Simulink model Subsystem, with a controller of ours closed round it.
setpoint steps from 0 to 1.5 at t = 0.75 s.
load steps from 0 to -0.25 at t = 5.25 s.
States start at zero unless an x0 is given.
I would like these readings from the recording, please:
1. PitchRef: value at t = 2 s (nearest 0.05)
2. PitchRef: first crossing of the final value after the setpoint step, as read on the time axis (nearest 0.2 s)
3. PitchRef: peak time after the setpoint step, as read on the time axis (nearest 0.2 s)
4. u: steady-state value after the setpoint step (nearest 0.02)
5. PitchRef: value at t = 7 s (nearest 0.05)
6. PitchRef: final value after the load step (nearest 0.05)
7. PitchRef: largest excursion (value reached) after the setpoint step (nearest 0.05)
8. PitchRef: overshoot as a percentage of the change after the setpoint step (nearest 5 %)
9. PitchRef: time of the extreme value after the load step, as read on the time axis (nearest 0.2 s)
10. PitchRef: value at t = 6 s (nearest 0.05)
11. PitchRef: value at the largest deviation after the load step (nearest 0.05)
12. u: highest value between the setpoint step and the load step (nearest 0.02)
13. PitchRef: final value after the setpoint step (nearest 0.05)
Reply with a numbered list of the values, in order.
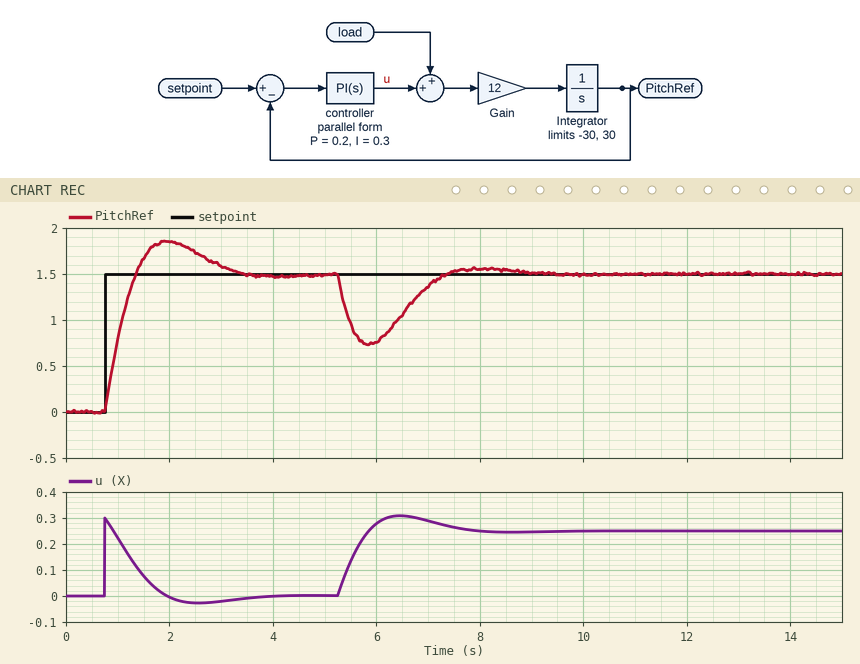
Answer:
1. 1.85
2. 1.4 s
3. 2.0 s
4. 0.00
5. 1.35
6. 1.50
7. 1.85
8. 25 %
9. 5.8 s
10. 0.75
11. 0.75
12. 0.30
13. 1.50
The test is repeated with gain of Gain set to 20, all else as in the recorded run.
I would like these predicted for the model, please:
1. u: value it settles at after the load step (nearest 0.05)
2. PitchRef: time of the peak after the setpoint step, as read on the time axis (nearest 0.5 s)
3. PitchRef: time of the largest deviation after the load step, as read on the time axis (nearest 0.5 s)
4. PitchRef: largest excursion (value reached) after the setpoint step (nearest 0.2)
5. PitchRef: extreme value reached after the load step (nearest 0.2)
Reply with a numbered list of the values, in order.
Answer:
1. 0.25
2. 1.5 s
3. 5.5 s
4. 1.8
5. 0.6
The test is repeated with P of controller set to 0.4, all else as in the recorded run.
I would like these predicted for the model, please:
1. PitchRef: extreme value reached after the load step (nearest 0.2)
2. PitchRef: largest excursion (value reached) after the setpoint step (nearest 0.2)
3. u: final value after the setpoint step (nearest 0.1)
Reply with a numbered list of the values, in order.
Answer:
1. 1.0
2. 1.6
3. 0.0
